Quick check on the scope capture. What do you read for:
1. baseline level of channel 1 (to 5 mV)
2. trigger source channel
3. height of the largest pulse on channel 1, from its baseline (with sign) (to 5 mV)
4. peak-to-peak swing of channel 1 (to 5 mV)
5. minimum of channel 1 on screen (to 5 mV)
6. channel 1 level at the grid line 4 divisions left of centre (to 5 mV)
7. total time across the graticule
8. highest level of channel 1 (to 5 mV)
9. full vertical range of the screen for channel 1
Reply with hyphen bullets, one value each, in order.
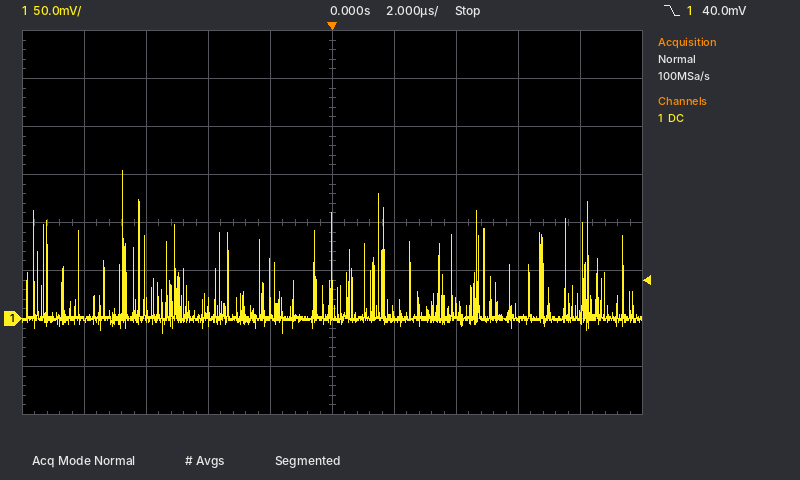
- 0 mV
- channel 1
- +155 mV
- 170 mV
- -15 mV
- 0 mV
- 20 µs
- 155 mV
- 400 mV
